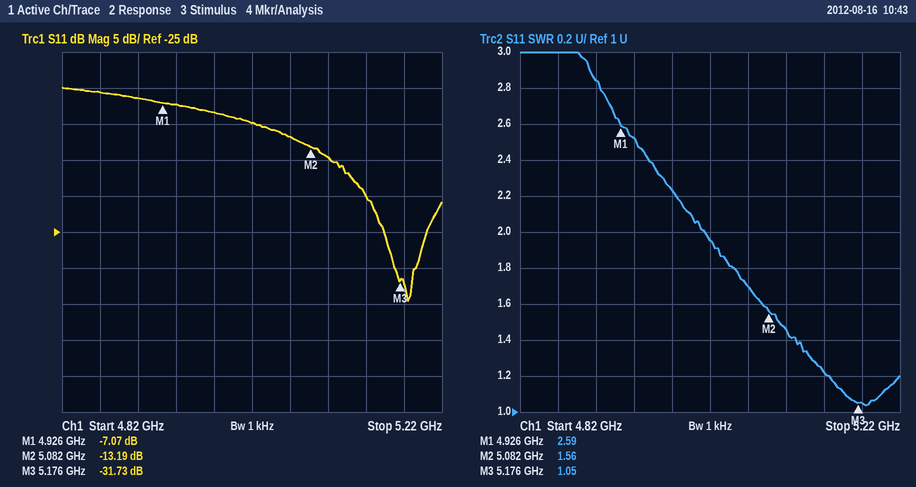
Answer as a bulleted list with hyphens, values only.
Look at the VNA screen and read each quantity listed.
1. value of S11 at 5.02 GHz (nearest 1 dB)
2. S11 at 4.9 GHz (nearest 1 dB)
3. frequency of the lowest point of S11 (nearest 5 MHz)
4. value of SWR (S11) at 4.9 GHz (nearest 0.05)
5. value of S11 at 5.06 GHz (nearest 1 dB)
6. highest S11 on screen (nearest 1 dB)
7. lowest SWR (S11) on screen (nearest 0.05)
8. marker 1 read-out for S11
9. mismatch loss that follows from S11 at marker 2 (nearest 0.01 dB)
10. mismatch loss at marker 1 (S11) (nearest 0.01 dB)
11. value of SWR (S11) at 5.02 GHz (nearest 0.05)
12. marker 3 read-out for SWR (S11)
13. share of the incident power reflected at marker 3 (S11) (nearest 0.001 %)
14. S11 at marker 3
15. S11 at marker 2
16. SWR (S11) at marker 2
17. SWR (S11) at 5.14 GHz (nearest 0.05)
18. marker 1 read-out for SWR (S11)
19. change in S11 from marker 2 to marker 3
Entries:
- -10 dB
- -6 dB
- 5.185 GHz
- 2.85
- -12 dB
- -5 dB
- 1.05
- -7.07 dB
- 0.21 dB
- 0.95 dB
- 1.95
- 1.05
- 0.067 %
- -31.73 dB
- -13.19 dB
- 1.56
- 1.20
- 2.59
- -18.54 dB
